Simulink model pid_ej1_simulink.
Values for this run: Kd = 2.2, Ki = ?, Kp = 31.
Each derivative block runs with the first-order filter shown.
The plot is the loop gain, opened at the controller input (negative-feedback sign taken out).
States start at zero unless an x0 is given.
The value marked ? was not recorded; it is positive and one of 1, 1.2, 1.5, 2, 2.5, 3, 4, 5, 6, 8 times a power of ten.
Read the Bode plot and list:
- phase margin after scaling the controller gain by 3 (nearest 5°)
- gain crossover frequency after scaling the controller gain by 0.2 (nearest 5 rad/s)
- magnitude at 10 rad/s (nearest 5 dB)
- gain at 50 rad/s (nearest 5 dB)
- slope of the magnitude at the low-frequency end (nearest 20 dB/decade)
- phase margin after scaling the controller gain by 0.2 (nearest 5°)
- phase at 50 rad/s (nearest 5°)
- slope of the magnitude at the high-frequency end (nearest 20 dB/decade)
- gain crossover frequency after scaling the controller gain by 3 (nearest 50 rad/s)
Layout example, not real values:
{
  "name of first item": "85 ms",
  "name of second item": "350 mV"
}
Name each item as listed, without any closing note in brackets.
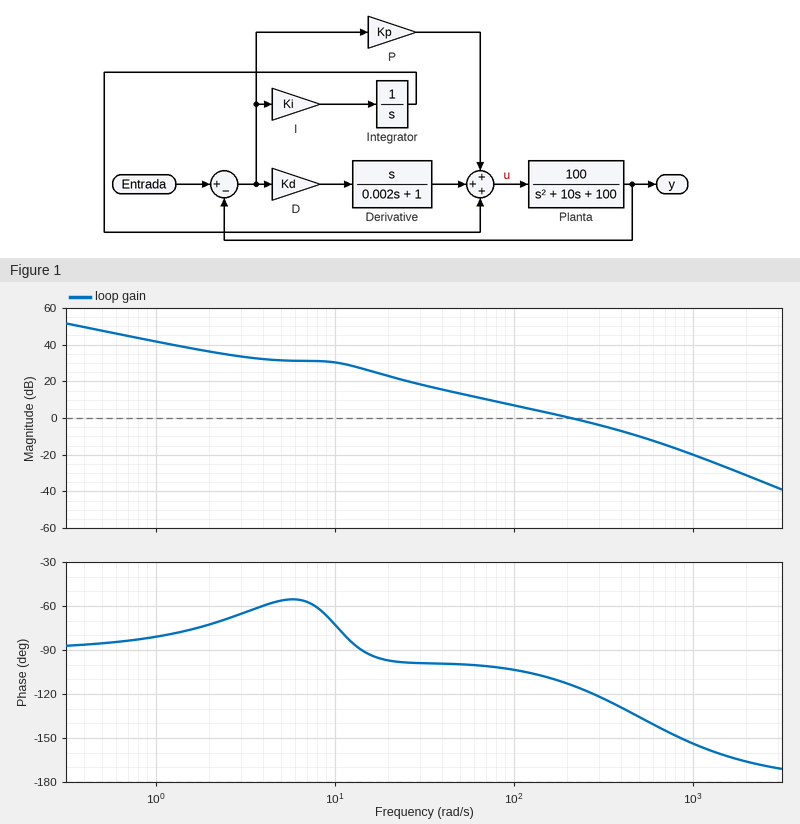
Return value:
{
  "phase margin after scaling the controller gain by 3": "45°",
  "gain crossover frequency after scaling the controller gain by 0.2": "45 rad/s",
  "magnitude at 10 rad/s": "30 dB",
  "gain at 50 rad/s": "15 dB",
  "slope of the magnitude at the low-frequency end": "-20 dB/decade",
  "phase margin after scaling the controller gain by 0.2": "80°",
  "phase at 50 rad/s": "-100°",
  "slope of the magnitude at the high-frequency end": "-40 dB/decade",
  "gain crossover frequency after scaling the controller gain by 3": "500 rad/s"
}
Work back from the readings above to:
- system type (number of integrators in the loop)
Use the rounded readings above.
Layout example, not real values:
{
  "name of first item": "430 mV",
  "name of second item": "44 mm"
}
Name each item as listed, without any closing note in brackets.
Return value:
{
  "system type": "1"
}
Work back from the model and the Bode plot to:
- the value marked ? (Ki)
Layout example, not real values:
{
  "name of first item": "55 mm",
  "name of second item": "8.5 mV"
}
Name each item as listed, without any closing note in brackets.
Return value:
{
  "the value marked ?": "120"
}
